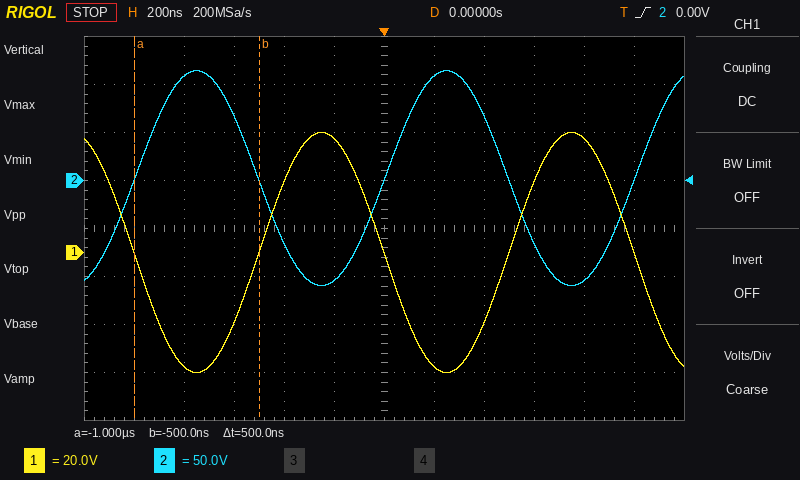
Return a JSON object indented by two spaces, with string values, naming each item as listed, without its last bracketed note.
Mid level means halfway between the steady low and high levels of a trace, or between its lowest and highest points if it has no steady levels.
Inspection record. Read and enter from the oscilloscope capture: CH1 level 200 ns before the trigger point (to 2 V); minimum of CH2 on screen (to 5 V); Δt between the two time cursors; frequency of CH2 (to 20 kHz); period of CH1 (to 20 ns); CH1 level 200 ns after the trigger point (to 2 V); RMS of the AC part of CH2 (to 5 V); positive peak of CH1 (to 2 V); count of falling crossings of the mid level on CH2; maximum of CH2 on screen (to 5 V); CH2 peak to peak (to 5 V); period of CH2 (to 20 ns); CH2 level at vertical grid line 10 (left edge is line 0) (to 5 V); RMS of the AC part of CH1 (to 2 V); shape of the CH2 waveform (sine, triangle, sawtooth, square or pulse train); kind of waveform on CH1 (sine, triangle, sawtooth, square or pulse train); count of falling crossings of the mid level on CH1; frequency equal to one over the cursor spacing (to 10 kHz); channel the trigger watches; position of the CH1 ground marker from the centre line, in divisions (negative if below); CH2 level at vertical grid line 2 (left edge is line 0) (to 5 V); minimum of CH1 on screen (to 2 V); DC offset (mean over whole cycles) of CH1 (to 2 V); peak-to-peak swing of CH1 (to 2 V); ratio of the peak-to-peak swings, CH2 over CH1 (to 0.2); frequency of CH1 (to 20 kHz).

{
  "CH1 level 200 ns before the trigger point": "48 V",
  "minimum of CH2 on screen": "-110 V",
  "Δt between the two time cursors": "500 ns",
  "frequency of CH2": "1.00 MHz",
  "period of CH1": "1.00 µs",
  "CH1 level 200 ns after the trigger point": "-48 V",
  "RMS of the AC part of CH2": "80 V",
  "positive peak of CH1": "50 V",
  "count of falling crossings of the mid level on CH2": "2",
  "maximum of CH2 on screen": "115 V",
  "CH2 peak to peak": "225 V",
  "period of CH2": "1.00 µs",
  "CH2 level at vertical grid line 10 (left edge is line 0)": "-105 V",
  "RMS of the AC part of CH1": "36 V",
  "shape of the CH2 waveform": "sine",
  "kind of waveform on CH1": "sine",
  "count of falling crossings of the mid level on CH1": "3",
  "frequency equal to one over the cursor spacing": "2.00 MHz",
  "channel the trigger watches": "CH2",
  "position of the CH1 ground marker from the centre line, in divisions": "-0.5 div",
  "CH2 level at vertical grid line 2 (left edge is line 0)": "110 V",
  "minimum of CH1 on screen": "-50 V",
  "DC offset (mean over whole cycles) of CH1": "0 V",
  "peak-to-peak swing of CH1": "100 V",
  "ratio of the peak-to-peak swings, CH2 over CH1": "2.2",
  "frequency of CH1": "1.00 MHz"
}
